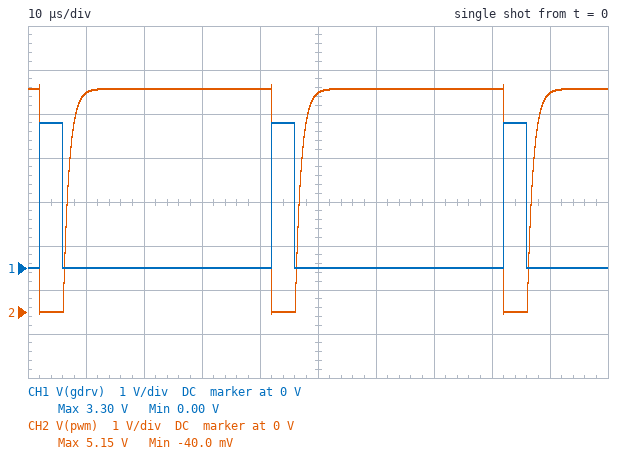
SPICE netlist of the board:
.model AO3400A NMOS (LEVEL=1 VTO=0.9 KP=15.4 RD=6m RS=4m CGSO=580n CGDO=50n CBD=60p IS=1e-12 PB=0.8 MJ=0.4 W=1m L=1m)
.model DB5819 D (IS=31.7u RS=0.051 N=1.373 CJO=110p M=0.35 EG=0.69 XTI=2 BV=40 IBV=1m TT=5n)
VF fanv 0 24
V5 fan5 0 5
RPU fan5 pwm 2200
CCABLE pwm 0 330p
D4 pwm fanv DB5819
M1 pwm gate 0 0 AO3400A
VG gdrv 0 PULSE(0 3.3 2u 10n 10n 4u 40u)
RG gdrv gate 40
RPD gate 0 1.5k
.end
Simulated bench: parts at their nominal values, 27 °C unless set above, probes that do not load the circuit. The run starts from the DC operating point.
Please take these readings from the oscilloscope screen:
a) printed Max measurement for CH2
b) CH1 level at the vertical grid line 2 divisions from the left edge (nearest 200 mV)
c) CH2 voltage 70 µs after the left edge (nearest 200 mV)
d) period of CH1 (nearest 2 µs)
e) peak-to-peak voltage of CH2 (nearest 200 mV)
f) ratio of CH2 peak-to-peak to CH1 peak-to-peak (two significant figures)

5.15 V
0 V
5.0 V
40 µs
5.2 V
1.6
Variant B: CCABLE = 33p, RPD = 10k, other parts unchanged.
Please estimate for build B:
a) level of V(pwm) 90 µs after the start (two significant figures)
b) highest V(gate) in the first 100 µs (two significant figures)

5.1 V
3.3 V
